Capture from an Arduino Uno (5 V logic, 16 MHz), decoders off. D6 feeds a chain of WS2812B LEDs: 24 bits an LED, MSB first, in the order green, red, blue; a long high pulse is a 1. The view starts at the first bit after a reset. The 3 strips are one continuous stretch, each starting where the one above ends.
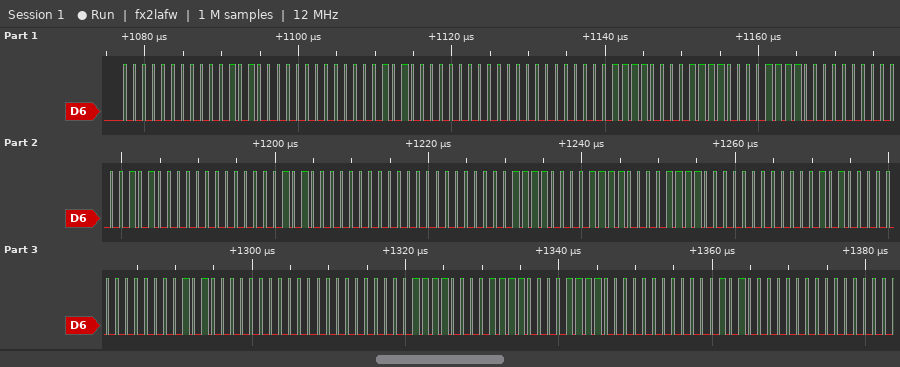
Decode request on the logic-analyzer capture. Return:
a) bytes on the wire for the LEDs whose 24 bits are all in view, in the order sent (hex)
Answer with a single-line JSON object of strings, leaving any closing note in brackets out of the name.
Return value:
{"bytes on the wire for the LEDs whose 24 bits are all in view, in the order sent": "00 14 00 14 00 00 1E 1E 1E 00 14 00 14 00 00 1E 1E 1E 00 14 00 14 00 00 1E 1E 1E 00 14 00"}
